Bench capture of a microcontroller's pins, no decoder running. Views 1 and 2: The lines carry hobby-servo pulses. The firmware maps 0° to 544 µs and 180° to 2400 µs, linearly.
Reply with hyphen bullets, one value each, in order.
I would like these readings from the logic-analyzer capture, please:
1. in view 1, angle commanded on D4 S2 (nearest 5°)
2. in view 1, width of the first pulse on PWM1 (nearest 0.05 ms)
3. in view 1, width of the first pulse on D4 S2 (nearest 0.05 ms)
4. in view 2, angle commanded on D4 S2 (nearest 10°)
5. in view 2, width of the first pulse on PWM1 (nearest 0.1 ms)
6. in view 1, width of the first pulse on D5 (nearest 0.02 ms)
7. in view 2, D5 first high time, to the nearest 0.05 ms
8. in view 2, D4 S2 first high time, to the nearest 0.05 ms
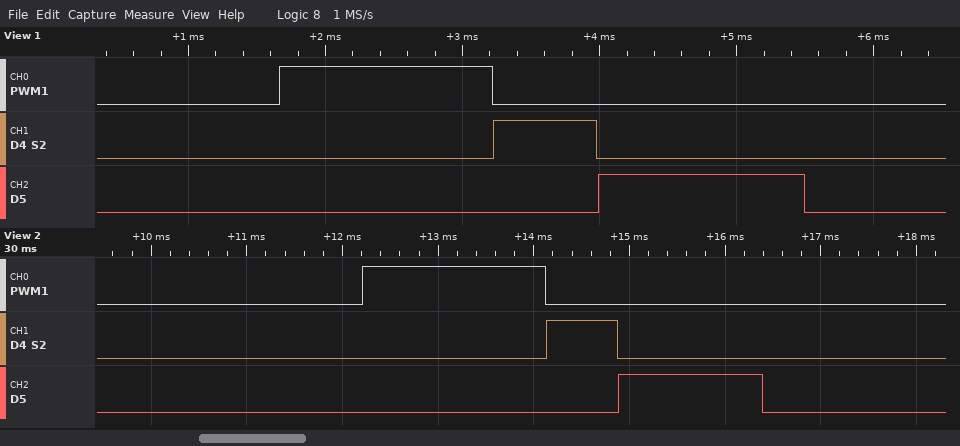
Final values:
- 20°
- 1.55 ms
- 0.75 ms
- 20°
- 1.9 ms
- 1.50 ms
- 1.50 ms
- 0.75 ms
